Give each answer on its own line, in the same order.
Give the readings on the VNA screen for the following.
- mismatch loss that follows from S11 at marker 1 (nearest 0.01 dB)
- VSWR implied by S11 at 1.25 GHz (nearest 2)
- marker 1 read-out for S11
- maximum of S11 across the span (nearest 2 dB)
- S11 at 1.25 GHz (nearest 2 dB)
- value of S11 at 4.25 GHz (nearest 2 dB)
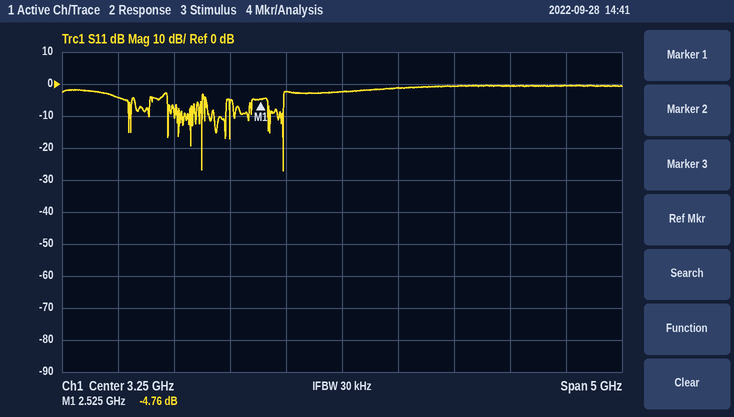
1.77 dB
4
-4.76 dB
0 dB
-4 dB
0 dB
